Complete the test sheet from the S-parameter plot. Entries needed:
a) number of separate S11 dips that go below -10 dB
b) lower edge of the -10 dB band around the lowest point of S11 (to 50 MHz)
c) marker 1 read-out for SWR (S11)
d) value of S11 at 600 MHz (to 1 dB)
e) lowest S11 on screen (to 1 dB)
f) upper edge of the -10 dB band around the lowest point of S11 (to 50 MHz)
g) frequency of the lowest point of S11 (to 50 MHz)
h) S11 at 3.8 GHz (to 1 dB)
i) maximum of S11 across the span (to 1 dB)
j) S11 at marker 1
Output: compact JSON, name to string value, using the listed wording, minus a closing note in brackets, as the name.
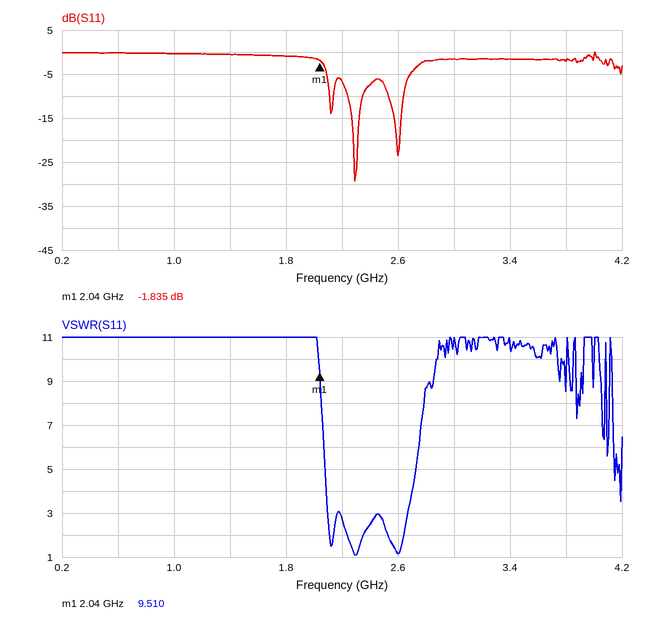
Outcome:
{"number of separate S11 dips that go below -10 dB": "3", "lower edge of the -10 dB band around the lowest point of S11": "2.25 GHz", "marker 1 read-out for SWR": "9.510", "value of S11 at 600 MHz": "0 dB", "lowest S11 on screen": "-29 dB", "upper edge of the -10 dB band around the lowest point of S11": "2.35 GHz", "frequency of the lowest point of S11": "2.30 GHz", "S11 at 3.8 GHz": "-2 dB", "maximum of S11 across the span": "0 dB", "S11 at marker 1": "-1.835 dB"}
